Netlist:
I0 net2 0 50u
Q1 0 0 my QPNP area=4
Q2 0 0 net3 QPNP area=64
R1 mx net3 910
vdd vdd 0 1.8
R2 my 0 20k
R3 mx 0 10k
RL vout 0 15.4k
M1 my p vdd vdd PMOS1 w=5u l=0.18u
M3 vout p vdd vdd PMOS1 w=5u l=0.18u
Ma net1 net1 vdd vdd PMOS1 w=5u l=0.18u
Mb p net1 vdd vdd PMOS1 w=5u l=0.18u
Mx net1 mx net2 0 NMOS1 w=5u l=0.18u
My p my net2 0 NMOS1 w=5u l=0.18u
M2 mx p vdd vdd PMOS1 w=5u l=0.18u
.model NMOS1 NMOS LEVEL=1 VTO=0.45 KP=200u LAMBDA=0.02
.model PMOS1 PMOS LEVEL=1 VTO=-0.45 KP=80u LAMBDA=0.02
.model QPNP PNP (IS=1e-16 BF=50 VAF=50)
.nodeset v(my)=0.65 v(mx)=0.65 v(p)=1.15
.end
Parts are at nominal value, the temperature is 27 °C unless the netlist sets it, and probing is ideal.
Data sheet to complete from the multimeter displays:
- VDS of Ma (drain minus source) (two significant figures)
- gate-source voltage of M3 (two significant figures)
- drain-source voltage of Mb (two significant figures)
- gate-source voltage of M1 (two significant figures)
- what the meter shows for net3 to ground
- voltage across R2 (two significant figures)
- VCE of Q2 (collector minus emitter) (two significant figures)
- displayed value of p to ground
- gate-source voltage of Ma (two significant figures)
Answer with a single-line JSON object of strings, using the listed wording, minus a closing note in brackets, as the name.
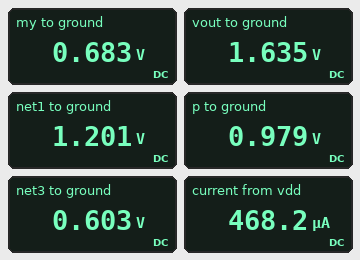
{"VDS of Ma (drain minus source)": "-600 mV", "gate-source voltage of M3": "-820 mV", "drain-source voltage of Mb": "-820 mV", "gate-source voltage of M1": "-820 mV", "what the meter shows for net3 to ground": "0.603 V", "voltage across R2": "680 mV", "VCE of Q2 (collector minus emitter)": "-600 mV", "displayed value of p to ground": "0.979 V", "gate-source voltage of Ma": "-600 mV"}
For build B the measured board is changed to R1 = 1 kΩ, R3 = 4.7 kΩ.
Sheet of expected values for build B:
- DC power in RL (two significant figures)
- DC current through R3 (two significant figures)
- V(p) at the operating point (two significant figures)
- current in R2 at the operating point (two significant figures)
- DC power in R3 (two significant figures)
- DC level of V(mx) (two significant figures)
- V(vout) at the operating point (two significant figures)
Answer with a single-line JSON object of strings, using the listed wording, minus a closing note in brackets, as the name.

{"DC power in RL": "180 µW", "DC current through R3": "150 µA", "V(p) at the operating point": "890 mV", "current in R2 at the operating point": "35 µA", "DC power in R3": "100 µW", "DC level of V(mx)": "700 mV", "V(vout) at the operating point": "1.7 V"}
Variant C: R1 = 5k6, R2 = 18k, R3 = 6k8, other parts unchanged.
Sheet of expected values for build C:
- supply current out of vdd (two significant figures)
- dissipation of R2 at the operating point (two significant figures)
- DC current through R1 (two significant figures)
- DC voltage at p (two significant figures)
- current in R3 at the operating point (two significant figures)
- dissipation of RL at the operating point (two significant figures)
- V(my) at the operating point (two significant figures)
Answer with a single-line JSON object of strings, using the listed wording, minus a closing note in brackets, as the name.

{"supply current out of vdd": "390 µA", "dissipation of R2 at the operating point": "25 µW", "DC current through R1": "19 µA", "DC voltage at p": "1.0 V", "current in R3 at the operating point": "99 µA", "dissipation of RL at the operating point": "160 µW", "V(my) at the operating point": "670 mV"}
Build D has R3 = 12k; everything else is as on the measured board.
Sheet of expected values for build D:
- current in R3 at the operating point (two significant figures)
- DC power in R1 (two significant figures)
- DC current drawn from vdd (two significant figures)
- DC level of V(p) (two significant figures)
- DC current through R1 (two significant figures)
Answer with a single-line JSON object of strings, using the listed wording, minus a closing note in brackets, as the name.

{"current in R3 at the operating point": "57 µA", "DC power in R1": "6.6 µW", "DC current drawn from vdd": "440 µA", "DC level of V(p)": "1.0 V", "DC current through R1": "85 µA"}
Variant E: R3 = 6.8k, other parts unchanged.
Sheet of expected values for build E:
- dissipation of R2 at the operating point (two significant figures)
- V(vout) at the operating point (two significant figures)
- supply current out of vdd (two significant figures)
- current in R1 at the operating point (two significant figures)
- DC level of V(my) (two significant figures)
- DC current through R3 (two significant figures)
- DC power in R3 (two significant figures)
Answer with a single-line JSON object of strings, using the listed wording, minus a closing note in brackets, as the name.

{"dissipation of R2 at the operating point": "24 µW", "V(vout) at the operating point": "1.7 V", "supply current out of vdd": "550 µA", "current in R1 at the operating point": "94 µA", "DC level of V(my)": "690 mV", "DC current through R3": "100 µA", "DC power in R3": "70 µW"}
